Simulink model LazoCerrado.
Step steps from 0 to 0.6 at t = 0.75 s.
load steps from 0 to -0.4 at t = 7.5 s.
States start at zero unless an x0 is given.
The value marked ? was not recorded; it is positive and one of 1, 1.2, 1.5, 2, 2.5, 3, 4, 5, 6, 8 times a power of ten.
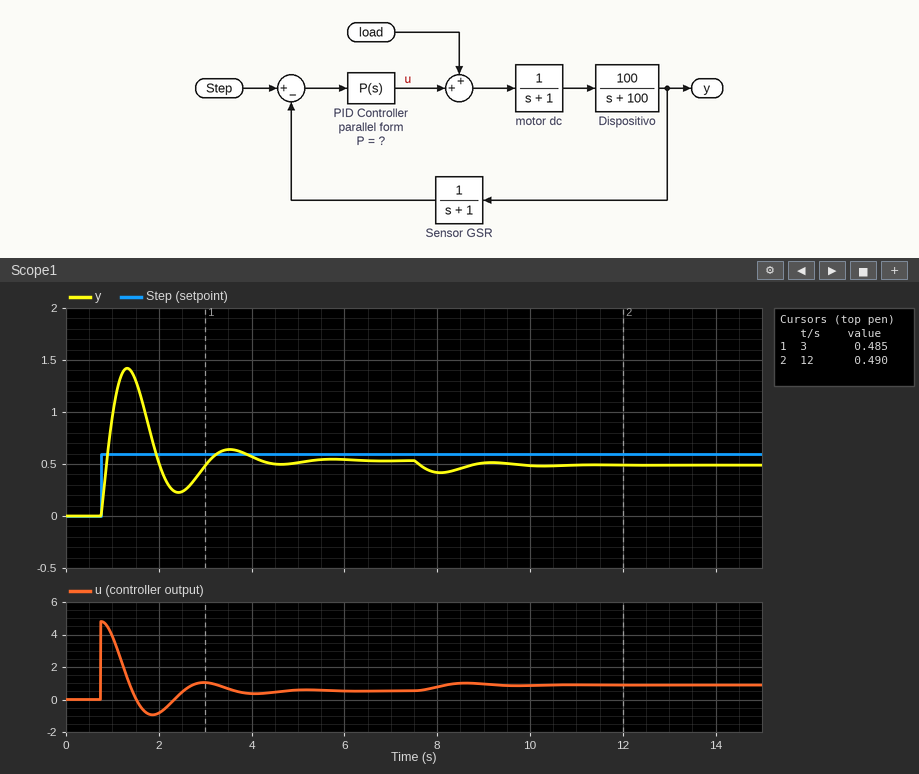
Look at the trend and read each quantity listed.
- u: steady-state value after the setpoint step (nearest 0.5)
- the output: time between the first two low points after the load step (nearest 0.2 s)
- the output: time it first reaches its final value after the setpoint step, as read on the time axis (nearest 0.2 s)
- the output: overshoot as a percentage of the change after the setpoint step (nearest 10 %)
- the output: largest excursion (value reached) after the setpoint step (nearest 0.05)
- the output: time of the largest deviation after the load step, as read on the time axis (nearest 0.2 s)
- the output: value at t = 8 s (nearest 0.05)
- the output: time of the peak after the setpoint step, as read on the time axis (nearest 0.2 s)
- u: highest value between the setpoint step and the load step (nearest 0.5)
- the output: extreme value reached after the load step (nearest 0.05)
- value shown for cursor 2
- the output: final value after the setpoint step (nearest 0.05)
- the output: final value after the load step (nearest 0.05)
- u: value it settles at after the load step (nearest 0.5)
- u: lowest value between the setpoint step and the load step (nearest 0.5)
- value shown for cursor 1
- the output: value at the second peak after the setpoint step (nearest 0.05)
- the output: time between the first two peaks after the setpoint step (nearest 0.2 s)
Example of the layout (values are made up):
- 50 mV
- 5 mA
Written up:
- 0.5
- 2.2 s
- 0.8 s
- 170 %
- 1.40
- 8.0 s
- 0.40
- 1.4 s
- 5.0
- 0.40
- 0.490
- 0.55
- 0.50
- 1.0
- -1.0
- 0.485
- 0.65
- 2.2 s
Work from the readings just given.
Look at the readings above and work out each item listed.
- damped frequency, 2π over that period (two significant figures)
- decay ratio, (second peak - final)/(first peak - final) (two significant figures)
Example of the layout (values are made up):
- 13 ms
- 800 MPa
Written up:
- 2.9 rad/s
- 0.12
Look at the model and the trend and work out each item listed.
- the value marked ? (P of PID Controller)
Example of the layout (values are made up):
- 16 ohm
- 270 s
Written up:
- 8
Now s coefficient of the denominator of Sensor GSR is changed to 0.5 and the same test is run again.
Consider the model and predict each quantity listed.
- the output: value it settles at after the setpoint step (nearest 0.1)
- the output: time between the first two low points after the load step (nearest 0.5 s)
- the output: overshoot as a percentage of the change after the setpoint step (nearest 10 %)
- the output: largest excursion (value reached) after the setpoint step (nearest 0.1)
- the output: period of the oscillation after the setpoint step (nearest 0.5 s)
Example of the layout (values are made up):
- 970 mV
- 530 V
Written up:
- 0.5
- 1.5 s
- 110 %
- 1.1
- 1.5 s
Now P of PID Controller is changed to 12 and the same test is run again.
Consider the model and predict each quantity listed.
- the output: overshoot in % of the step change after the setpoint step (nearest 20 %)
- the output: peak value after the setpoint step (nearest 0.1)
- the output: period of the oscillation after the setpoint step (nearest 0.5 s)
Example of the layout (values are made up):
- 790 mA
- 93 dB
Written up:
- 220 %
- 1.8
- 2.0 s
